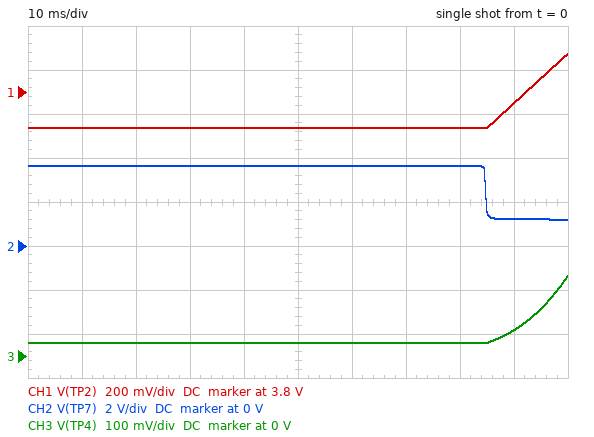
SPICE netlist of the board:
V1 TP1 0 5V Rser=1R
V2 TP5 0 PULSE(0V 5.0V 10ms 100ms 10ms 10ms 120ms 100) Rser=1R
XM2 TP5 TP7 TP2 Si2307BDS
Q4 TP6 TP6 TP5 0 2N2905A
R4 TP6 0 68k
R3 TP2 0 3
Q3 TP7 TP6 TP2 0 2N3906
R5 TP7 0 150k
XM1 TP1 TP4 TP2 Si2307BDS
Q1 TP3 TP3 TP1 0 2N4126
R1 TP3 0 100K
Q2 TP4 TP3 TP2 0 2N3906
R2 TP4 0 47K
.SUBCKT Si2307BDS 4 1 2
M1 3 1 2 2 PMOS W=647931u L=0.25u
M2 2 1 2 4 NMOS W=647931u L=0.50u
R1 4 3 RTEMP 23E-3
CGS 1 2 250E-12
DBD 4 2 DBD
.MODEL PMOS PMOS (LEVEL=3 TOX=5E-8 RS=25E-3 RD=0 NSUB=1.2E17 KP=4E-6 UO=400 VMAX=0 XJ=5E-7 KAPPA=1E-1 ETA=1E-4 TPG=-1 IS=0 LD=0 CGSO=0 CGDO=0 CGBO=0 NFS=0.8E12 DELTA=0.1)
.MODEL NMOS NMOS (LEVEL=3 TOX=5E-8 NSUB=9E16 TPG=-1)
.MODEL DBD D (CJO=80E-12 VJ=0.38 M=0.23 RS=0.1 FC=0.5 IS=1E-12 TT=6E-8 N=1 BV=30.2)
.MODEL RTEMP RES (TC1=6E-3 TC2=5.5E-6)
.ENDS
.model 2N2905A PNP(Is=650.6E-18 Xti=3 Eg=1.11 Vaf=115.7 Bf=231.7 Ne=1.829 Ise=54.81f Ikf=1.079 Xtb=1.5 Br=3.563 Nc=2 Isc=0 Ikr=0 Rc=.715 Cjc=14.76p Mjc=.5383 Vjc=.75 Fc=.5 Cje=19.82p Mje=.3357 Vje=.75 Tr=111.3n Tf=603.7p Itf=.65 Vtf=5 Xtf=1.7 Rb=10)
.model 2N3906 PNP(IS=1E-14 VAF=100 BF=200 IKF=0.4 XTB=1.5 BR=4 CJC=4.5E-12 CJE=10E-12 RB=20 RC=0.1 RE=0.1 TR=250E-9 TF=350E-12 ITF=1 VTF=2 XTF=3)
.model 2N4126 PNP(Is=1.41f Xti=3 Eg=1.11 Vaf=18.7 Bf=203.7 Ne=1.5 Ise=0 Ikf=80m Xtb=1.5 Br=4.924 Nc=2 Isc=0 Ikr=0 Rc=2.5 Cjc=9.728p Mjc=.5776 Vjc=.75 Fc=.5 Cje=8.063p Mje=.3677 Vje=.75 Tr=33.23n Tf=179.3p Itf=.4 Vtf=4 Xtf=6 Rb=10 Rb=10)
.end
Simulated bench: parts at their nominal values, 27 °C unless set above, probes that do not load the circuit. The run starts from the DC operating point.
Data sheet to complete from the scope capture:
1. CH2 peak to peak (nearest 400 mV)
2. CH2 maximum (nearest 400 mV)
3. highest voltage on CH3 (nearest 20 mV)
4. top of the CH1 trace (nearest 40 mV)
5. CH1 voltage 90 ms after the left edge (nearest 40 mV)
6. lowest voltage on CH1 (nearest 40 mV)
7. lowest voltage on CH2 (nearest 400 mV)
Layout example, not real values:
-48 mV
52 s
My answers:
2.4 V
3.6 V
180 mV
3.96 V
3.76 V
3.64 V
1.2 V
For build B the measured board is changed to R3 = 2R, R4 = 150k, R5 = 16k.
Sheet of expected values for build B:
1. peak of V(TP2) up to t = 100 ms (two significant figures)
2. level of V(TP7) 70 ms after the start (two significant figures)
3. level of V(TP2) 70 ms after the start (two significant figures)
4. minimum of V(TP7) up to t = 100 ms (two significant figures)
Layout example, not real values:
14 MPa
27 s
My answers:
3.7 V
3.1 V
3.2 V
150 mV
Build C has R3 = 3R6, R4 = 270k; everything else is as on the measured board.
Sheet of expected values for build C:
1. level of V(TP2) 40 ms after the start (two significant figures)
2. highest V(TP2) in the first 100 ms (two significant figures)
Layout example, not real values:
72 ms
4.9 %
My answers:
3.8 V
4.1 V
